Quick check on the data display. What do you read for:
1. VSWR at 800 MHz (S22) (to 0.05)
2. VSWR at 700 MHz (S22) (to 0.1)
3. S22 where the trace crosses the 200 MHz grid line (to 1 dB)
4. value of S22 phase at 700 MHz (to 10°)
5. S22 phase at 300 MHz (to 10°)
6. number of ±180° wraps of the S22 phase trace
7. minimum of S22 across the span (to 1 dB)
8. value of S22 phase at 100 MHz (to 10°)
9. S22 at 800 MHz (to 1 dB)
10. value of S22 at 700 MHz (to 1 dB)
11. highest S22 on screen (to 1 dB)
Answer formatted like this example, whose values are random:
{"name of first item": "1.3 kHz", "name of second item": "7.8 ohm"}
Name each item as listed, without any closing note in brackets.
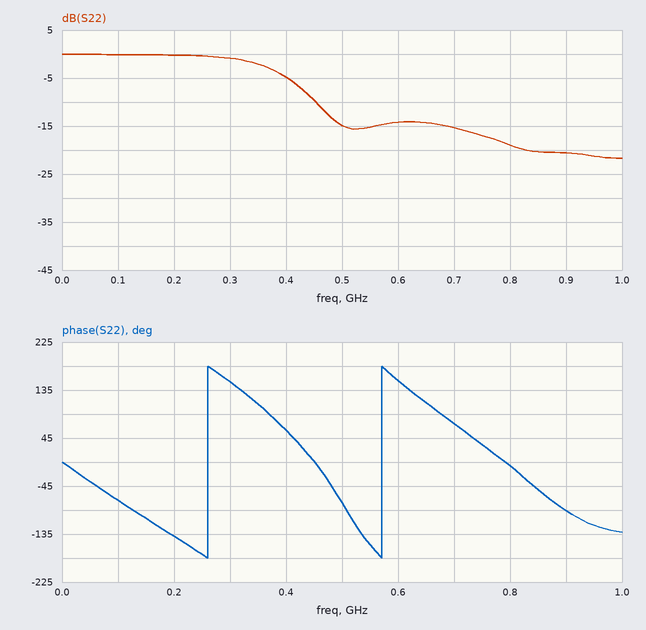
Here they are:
{"VSWR at 800 MHz (S22)": "1.25", "VSWR at 700 MHz (S22)": "1.4", "S22 where the trace crosses the 200 MHz grid line": "0 dB", "value of S22 phase at 700 MHz": "70°", "S22 phase at 300 MHz": "150°", "number of ±180° wraps of the S22 phase trace": "2", "minimum of S22 across the span": "-22 dB", "value of S22 phase at 100 MHz": "-70°", "S22 at 800 MHz": "-19 dB", "value of S22 at 700 MHz": "-15 dB", "highest S22 on screen": "0 dB"}
